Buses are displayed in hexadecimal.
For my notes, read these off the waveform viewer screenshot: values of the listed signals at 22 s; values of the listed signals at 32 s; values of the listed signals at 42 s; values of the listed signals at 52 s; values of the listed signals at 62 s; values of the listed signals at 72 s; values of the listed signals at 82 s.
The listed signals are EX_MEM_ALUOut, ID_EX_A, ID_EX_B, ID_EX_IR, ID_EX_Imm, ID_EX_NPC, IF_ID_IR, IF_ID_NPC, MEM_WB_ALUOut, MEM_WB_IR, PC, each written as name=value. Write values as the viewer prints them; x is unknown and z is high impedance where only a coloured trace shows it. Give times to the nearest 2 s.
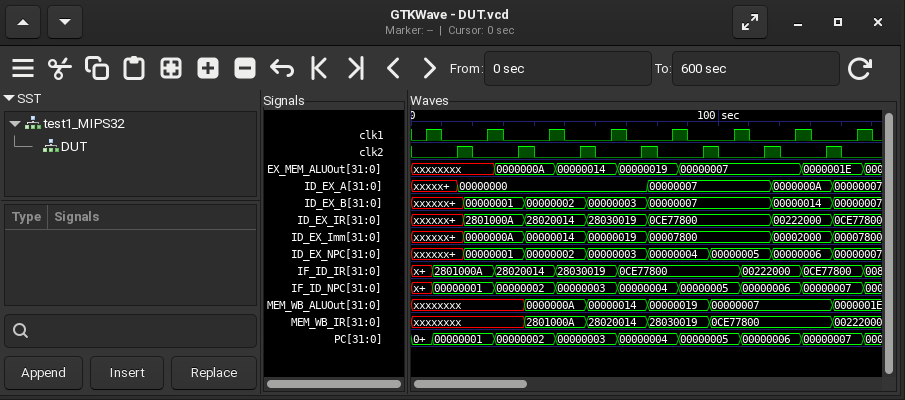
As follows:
EX_MEM_ALUOut=xxxxxxxx, ID_EX_A=00000000, ID_EX_B=00000001, ID_EX_IR=2801000A, ID_EX_Imm=0000000A, ID_EX_NPC=00000001, IF_ID_IR=2801000A, IF_ID_NPC=00000001, MEM_WB_ALUOut=xxxxxxxx, MEM_WB_IR=xxxxxxxx, PC=00000001
EX_MEM_ALUOut=0000000A, ID_EX_A=00000000, ID_EX_B=00000001, ID_EX_IR=2801000A, ID_EX_Imm=0000000A, ID_EX_NPC=00000001, IF_ID_IR=28020014, IF_ID_NPC=00000002, MEM_WB_ALUOut=xxxxxxxx, MEM_WB_IR=xxxxxxxx, PC=00000002
EX_MEM_ALUOut=0000000A, ID_EX_A=00000000, ID_EX_B=00000002, ID_EX_IR=28020014, ID_EX_Imm=00000014, ID_EX_NPC=00000002, IF_ID_IR=28020014, IF_ID_NPC=00000002, MEM_WB_ALUOut=0000000A, MEM_WB_IR=2801000A, PC=00000002
EX_MEM_ALUOut=00000014, ID_EX_A=00000000, ID_EX_B=00000002, ID_EX_IR=28020014, ID_EX_Imm=00000014, ID_EX_NPC=00000002, IF_ID_IR=28030019, IF_ID_NPC=00000003, MEM_WB_ALUOut=0000000A, MEM_WB_IR=2801000A, PC=00000003
EX_MEM_ALUOut=00000014, ID_EX_A=00000000, ID_EX_B=00000003, ID_EX_IR=28030019, ID_EX_Imm=00000019, ID_EX_NPC=00000003, IF_ID_IR=28030019, IF_ID_NPC=00000003, MEM_WB_ALUOut=00000014, MEM_WB_IR=28020014, PC=00000003
EX_MEM_ALUOut=00000019, ID_EX_A=00000000, ID_EX_B=00000003, ID_EX_IR=28030019, ID_EX_Imm=00000019, ID_EX_NPC=00000003, IF_ID_IR=0CE77800, IF_ID_NPC=00000004, MEM_WB_ALUOut=00000014, MEM_WB_IR=28020014, PC=00000004
EX_MEM_ALUOut=00000019, ID_EX_A=00000007, ID_EX_B=00000007, ID_EX_IR=0CE77800, ID_EX_Imm=00007800, ID_EX_NPC=00000004, IF_ID_IR=0CE77800, IF_ID_NPC=00000004, MEM_WB_ALUOut=00000019, MEM_WB_IR=28030019, PC=00000004
